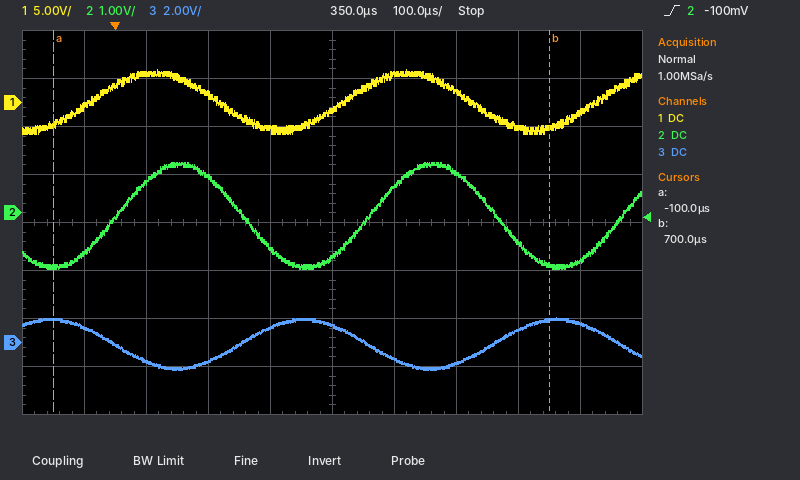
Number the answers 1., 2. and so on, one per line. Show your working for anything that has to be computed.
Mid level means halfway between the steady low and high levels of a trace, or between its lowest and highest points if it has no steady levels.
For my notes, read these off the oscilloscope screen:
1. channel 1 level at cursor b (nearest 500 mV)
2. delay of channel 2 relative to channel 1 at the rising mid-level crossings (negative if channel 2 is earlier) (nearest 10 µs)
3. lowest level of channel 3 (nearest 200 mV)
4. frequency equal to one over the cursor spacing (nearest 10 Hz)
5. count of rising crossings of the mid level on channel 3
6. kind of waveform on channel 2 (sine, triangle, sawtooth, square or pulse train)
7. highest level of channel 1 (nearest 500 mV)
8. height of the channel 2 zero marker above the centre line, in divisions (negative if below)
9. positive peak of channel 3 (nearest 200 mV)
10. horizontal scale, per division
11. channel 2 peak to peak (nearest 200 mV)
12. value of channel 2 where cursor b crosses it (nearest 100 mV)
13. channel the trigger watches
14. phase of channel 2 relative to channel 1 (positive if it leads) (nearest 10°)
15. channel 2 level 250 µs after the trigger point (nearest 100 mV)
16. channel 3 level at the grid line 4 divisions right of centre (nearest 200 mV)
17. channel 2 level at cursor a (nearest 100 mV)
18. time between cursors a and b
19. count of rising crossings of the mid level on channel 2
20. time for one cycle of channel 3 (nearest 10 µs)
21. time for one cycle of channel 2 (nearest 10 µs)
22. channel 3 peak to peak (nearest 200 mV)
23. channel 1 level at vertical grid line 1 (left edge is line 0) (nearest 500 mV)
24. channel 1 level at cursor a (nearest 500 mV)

1. -2.5 V
2. +40 µs
3. -1.2 V
4. 1 / 800 µs ≈ 1.25 kHz
5. 2
6. sine
7. 3.5 V
8. +0.2 div
9. 1.0 V
10. 100 µs
11. 2.2 V
12. -1.1 V
13. channel 2
14. −360° × (+40 µs) / 410 µs ≈ -35.1°, so -40° to the nearest 10°
15. -700 mV
16. 800 mV
17. -1.1 V
18. 700 µs − (-100 µs) = 800 µs
19. 3
20. 410 µs
21. 410 µs
22. 1.0 V − (-1.2 V) = 2.2 V
23. -500 mV
24. -2.0 V
